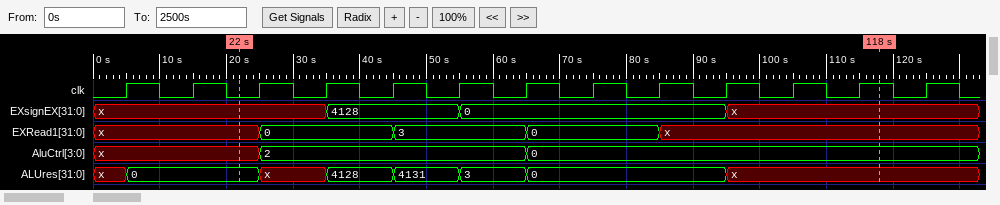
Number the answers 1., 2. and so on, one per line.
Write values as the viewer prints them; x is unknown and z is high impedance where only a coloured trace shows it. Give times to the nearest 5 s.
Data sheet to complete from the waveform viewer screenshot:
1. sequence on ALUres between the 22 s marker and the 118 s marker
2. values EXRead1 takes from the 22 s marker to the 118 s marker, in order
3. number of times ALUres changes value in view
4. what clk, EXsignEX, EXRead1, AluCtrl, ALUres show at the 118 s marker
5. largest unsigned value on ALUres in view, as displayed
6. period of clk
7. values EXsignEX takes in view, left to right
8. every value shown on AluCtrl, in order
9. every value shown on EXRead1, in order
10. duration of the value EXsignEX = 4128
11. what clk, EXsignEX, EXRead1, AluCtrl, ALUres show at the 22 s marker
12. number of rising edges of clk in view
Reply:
1. 0, x, 4128, 4131, 3, 0, x
2. x, 0, 3, 0, x
3. 7
4. clk=1, EXsignEX=x, EXRead1=x, AluCtrl=0, ALUres=x
5. 4131
6. 10 s
7. x, 4128, 0, x
8. x, 2, 0
9. x, 0, 3, 0, x
10. 20 s
11. clk=0, EXsignEX=x, EXRead1=x, AluCtrl=x, ALUres=0
12. 13
